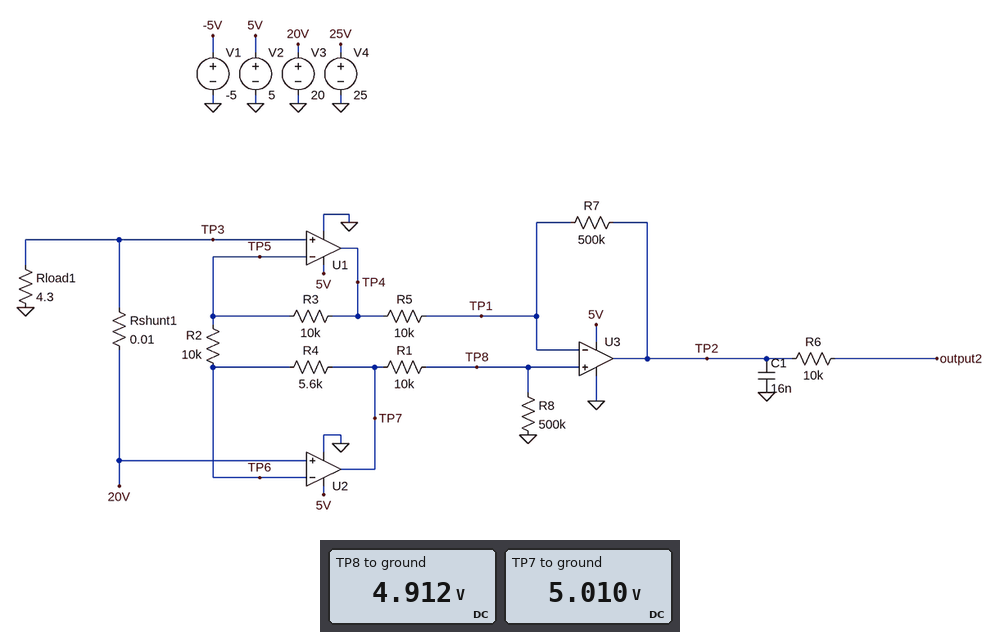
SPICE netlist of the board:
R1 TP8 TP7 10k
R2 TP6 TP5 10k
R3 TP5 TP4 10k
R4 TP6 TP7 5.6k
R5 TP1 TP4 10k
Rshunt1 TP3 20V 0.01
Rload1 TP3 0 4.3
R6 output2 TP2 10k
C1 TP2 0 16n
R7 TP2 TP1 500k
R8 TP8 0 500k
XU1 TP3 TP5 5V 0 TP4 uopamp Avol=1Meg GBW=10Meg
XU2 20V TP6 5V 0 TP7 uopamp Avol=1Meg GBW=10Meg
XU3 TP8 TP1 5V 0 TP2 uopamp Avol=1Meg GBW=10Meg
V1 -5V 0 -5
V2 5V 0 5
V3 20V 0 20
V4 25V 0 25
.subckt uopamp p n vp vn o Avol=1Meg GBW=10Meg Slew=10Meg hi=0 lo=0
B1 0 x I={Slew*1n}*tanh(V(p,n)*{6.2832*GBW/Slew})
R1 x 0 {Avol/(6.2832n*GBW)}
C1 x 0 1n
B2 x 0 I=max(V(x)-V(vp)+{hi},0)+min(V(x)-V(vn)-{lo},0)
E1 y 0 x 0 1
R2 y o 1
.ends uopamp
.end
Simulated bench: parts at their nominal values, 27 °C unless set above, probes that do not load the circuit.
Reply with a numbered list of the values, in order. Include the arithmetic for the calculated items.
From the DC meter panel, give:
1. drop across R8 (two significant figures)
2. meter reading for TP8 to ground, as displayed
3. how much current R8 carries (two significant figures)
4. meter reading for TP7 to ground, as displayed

1. 4.912 V = 4.9 V
2. 4.912 V
3. (4.912 V) / 500 kΩ = 9.8 µA
4. 5.010 V
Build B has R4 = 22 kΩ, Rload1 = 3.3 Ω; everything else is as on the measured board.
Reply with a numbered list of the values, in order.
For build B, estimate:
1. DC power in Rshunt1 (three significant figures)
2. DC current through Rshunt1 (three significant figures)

1. 365 mW
2. 6.04 A
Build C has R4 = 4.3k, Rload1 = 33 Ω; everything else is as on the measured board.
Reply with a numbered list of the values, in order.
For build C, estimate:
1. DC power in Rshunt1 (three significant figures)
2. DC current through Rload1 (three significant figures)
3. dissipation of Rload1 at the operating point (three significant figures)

1. 3.67 mW
2. 606 mA
3. 12.1 W
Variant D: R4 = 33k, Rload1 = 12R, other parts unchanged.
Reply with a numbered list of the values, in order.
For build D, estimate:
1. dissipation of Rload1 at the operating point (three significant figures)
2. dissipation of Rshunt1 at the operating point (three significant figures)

1. 33.3 W
2. 27.7 mW
